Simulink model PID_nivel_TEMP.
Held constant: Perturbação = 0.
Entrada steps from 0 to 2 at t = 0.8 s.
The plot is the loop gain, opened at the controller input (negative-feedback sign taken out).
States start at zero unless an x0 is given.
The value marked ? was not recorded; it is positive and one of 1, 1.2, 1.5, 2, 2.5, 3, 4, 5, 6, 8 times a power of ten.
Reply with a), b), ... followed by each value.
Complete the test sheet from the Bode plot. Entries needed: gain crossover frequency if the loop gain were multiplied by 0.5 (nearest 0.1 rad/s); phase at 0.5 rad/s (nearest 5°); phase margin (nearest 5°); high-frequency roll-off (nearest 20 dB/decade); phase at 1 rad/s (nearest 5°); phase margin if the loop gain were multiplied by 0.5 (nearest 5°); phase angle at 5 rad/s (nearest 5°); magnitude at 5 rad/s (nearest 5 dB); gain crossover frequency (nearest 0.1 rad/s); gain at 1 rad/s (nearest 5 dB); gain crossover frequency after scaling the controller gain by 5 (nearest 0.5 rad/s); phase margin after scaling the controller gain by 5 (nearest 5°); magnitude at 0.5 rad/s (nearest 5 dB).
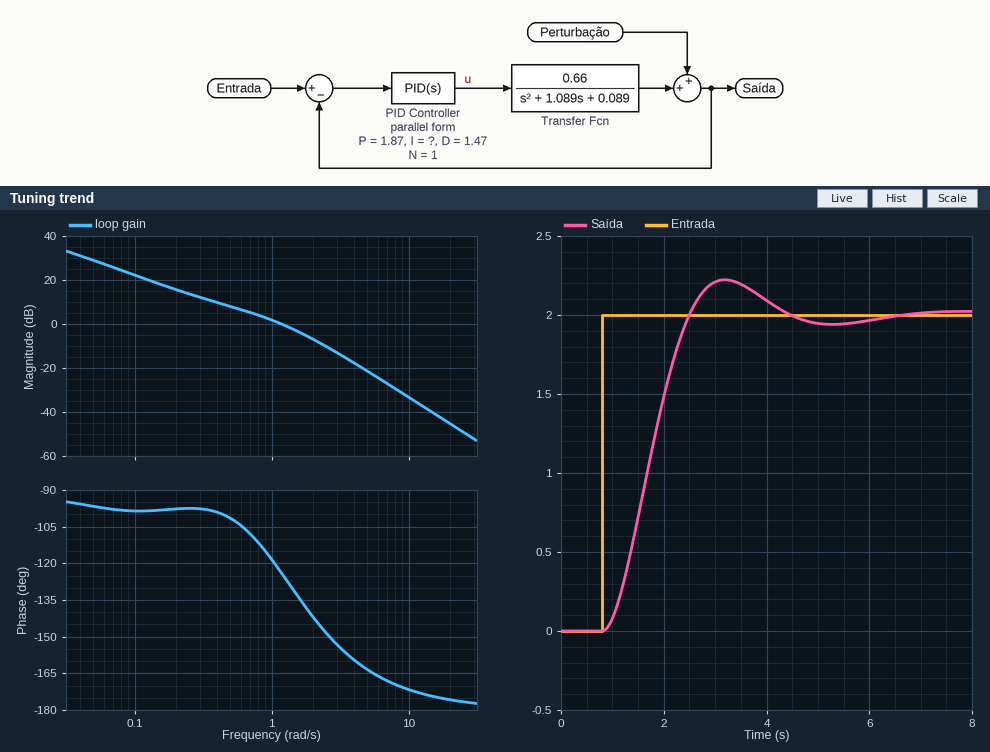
a) 0.6 rad/s
b) -100°
c) 55°
d) -40 dB/decade
e) -120°
f) 75°
g) -165°
h) -20 dB
i) 1.2 rad/s
j) 0 dB
k) 3.0 rad/s
l) 25°
m) 10 dB
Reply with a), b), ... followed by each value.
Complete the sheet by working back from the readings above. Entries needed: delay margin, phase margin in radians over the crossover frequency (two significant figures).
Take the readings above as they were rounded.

a) 0.80 s
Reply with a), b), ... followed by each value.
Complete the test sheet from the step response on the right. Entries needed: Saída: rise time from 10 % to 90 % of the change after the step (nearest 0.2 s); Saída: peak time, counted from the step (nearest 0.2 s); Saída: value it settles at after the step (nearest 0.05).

a) 1.2 s
b) 2.4 s
c) 2.00
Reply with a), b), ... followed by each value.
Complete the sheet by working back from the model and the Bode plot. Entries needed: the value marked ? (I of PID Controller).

a) 0.2
